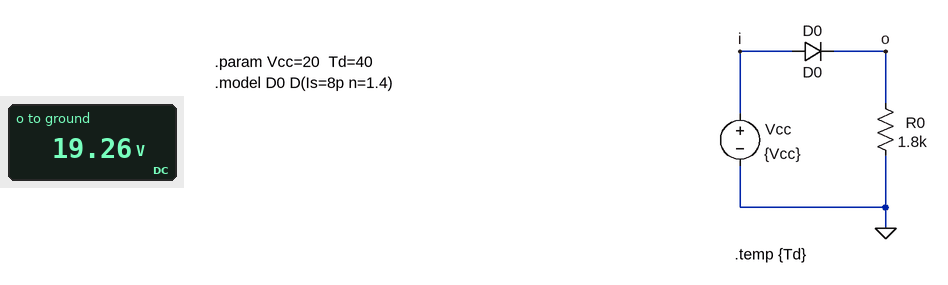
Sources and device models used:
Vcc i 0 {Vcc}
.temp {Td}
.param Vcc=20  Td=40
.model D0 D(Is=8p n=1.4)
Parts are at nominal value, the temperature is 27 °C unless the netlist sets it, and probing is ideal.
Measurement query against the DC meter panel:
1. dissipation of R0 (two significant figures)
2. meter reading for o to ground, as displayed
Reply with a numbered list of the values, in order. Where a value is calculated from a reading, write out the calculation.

1. (19.26 V)^2 / 1.8 kΩ = 210 mW
2. 19.26 V
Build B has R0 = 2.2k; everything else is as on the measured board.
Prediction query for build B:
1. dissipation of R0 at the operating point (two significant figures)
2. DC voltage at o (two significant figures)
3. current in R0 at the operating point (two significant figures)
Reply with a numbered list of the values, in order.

1. 170 mW
2. 19 V
3. 8.8 mA
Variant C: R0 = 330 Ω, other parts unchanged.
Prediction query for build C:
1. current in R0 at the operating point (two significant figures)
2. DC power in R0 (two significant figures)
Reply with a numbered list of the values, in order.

1. 58 mA
2. 1.1 W
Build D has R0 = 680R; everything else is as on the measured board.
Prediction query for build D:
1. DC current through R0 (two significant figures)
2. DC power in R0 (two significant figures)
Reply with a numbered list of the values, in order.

1. 28 mA
2. 540 mW
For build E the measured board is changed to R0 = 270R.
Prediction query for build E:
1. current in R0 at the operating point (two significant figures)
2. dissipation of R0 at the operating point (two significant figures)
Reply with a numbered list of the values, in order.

1. 71 mA
2. 1.4 W
